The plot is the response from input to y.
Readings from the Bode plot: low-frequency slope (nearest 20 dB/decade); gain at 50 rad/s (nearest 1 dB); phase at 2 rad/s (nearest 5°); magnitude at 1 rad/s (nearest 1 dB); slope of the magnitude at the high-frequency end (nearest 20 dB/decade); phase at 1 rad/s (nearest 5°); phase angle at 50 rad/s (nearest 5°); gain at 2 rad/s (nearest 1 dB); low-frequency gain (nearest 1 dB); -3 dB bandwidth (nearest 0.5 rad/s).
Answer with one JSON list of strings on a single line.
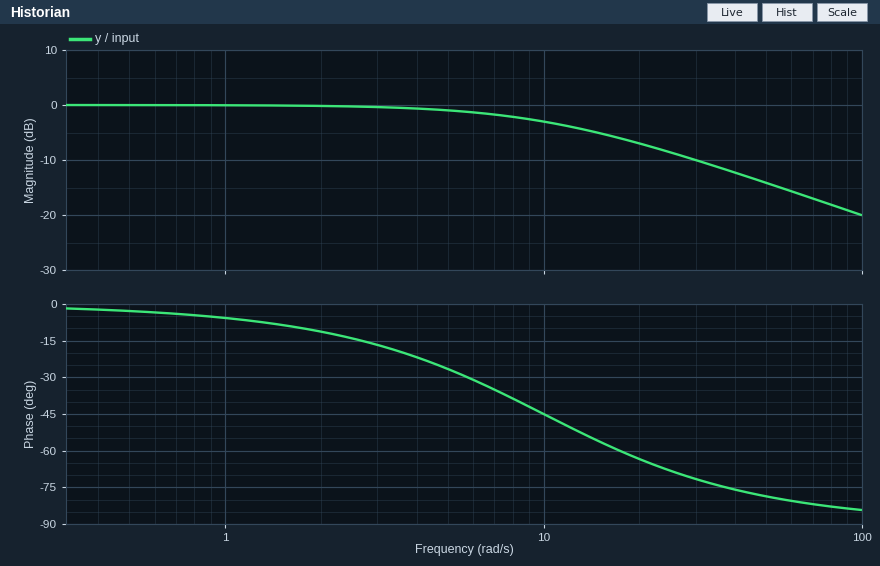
["0 dB/decade", "-14 dB", "-10°", "0 dB", "-20 dB/decade", "-5°", "-80°", "0 dB", "0 dB", "10.0 rad/s"]
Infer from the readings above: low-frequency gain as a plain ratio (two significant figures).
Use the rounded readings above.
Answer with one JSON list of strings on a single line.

["1.0"]
